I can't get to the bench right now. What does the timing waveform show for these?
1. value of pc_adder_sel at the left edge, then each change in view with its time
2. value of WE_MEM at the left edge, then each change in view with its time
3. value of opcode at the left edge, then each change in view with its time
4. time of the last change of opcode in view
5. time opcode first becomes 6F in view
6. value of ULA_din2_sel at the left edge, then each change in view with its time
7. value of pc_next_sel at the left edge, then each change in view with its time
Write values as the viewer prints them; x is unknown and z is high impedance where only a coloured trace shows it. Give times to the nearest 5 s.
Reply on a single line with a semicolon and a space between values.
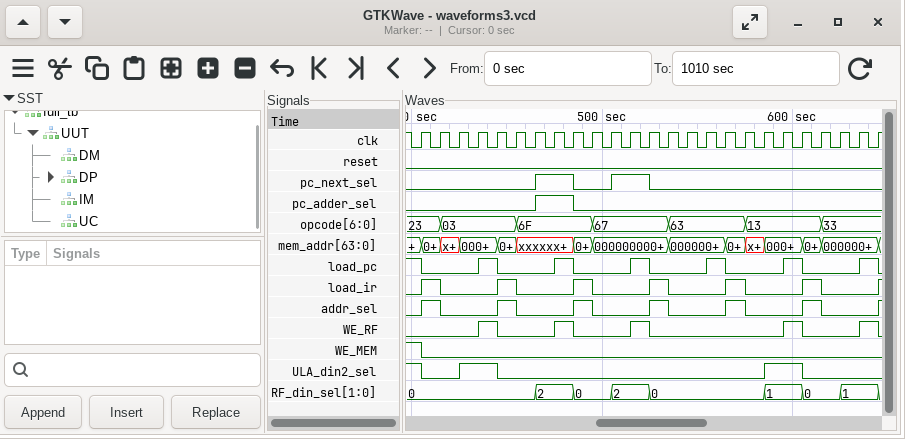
0, 1 at 465 s, 0 at 485 s; 1, 0 at 405 s; 23, 03 at 415 s, 6F at 455 s, 67 at 495 s, 63 at 535 s, 13 at 575 s, 33 at 615 s; 615 s; 455 s; 1, 0 at 405 s, 1 at 425 s, 0 at 445 s, 1 at 585 s, 0 at 605 s; 0, 1 at 465 s, 0 at 485 s, 1 at 505 s, 0 at 525 s
